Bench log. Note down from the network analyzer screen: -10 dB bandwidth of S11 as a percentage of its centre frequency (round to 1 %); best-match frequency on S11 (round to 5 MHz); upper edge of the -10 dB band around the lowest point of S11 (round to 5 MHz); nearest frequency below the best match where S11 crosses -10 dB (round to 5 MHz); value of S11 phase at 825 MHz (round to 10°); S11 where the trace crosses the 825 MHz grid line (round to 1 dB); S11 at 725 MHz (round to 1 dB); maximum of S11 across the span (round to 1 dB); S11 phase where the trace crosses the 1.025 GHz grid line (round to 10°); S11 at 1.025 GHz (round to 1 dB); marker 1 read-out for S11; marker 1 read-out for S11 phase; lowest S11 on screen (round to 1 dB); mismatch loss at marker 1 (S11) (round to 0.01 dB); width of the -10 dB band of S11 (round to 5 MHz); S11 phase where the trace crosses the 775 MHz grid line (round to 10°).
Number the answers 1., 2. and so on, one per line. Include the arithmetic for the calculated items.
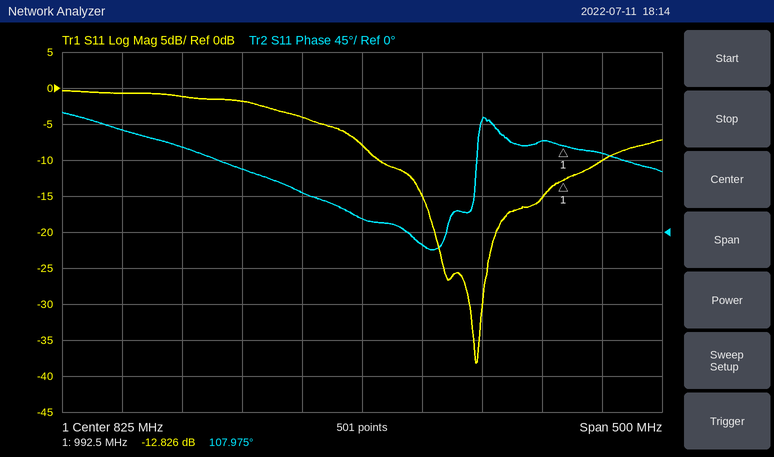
1. 185 MHz / 932.5 MHz ≈ 20 %
2. 920 MHz
3. 1.025 GHz
4. 840 MHz
5. 20°
6. -8 dB
7. -2 dB
8. 0 dB
9. 100°
10. -10 dB
11. -12.826 dB
12. 107.975°
13. -38 dB
14. −10 log10(1 − 10^(-12.826/10)) ≈ 0.23 dB
15. 1.025 GHz − 840 MHz = 185 MHz
16. 50°
